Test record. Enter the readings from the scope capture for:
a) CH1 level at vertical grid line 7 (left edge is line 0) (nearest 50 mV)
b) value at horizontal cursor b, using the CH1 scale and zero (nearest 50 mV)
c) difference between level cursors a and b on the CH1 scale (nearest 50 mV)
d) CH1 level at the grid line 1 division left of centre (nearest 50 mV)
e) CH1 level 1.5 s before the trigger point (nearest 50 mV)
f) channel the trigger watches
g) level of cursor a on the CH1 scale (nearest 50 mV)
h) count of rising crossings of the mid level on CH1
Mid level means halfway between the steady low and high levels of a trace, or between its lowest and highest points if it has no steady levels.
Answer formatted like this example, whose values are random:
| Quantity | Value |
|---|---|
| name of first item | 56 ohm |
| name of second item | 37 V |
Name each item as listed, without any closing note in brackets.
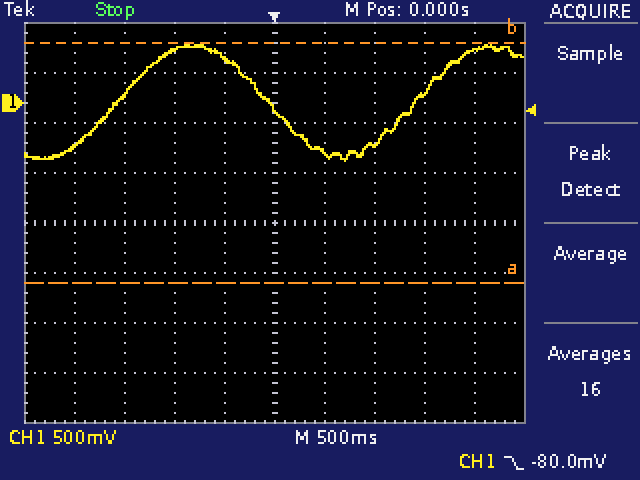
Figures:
| Quantity | Value |
|---|---|
| CH1 level at vertical grid line 7 (left edge is line 0) | -400 mV |
| value at horizontal cursor b, using the CH1 scale and zero | 600 mV |
| difference between level cursors a and b on the CH1 scale | 2.40 V |
| CH1 level at the grid line 1 division left of centre | 450 mV |
| CH1 level 1.5 s before the trigger point | 100 mV |
| channel the trigger watches | CH1 |
| level of cursor a on the CH1 scale | -1.80 V |
| count of rising crossings of the mid level on CH1 | 2 |
